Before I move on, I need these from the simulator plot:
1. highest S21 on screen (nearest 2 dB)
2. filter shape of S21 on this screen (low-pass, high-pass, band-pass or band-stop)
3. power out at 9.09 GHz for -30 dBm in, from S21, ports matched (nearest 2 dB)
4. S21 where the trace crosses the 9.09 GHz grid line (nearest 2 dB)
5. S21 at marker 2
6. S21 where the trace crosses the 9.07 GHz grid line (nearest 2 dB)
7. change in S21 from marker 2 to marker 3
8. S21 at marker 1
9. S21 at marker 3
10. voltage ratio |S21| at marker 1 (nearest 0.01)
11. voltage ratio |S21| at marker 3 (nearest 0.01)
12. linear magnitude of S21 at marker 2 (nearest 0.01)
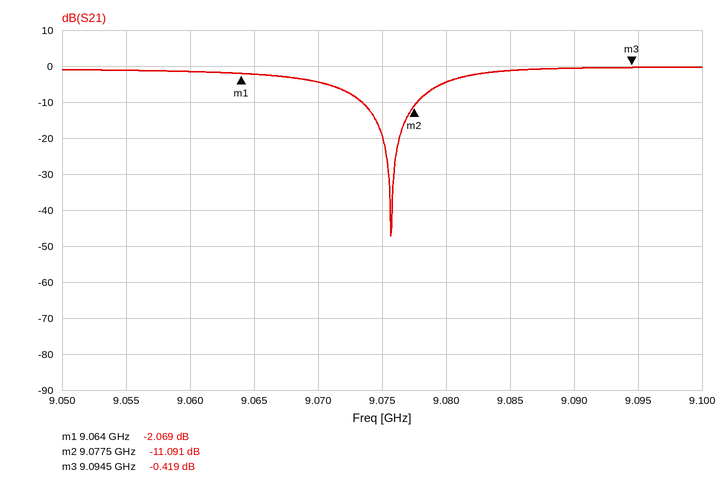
0 dB
band-stop
-30 dBm
0 dB
-11.091 dB
-4 dB
10.672 dB
-2.069 dB
-0.419 dB
0.79
0.95
0.28
